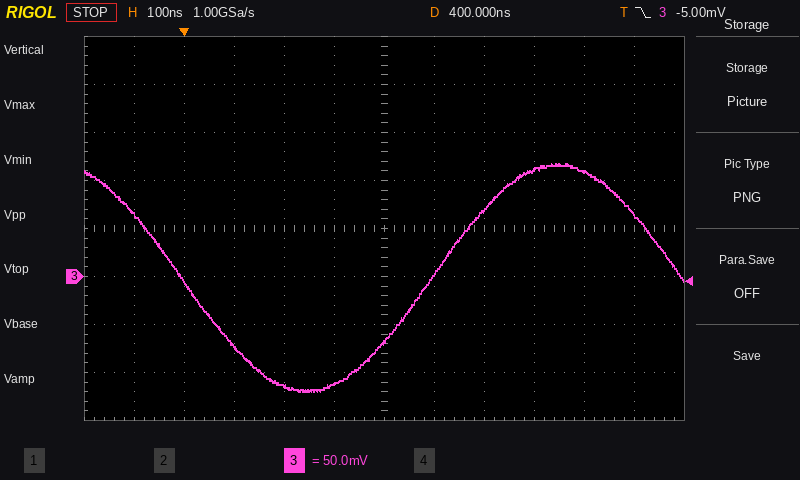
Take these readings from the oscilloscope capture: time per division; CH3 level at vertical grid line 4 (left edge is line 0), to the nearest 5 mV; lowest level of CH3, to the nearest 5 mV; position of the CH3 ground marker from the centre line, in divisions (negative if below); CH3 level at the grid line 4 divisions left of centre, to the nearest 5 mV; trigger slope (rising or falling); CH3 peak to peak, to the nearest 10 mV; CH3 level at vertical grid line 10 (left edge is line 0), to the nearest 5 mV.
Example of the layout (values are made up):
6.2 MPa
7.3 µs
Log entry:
100 ns
-115 mV
-120 mV
-1.0 div
-5 mV
falling
240 mV
110 mV
